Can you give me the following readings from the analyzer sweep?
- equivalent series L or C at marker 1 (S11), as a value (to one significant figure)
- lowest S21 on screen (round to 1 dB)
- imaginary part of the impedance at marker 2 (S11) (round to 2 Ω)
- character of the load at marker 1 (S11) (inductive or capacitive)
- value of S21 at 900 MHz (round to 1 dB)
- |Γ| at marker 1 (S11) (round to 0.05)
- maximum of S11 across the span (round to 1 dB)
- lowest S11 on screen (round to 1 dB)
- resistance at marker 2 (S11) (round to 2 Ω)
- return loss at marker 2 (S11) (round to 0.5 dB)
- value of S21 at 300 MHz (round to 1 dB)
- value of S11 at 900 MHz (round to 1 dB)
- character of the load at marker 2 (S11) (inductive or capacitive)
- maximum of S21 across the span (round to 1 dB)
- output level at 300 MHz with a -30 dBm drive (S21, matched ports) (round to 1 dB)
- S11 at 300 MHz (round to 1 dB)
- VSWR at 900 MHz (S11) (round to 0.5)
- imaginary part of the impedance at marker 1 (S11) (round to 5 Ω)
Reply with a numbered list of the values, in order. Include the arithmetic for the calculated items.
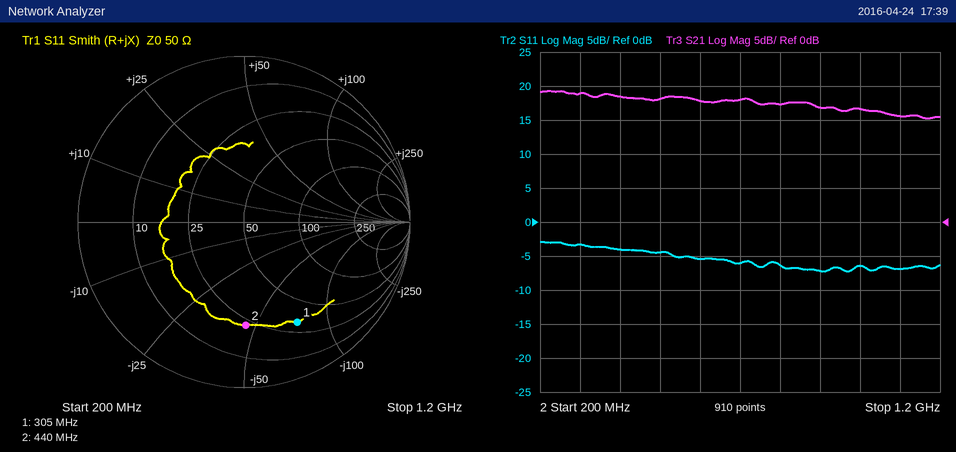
1. C = 1/(2π × 305 MHz × 75 Ω) ≈ 7 pF
2. 15 dB
3. -46 Ω
4. capacitive
5. 17 dB
6. 0.70
7. -3 dB
8. -7 dB
9. 22 Ω
10. 4.0 dB
11. 19 dB
12. -7 dB
13. capacitive
14. 19 dB
15. -30 dBm + (19 dB) = -11 dBm
16. -3 dB
17. |Γ| = 10^(-7/20) = 0.4467; VSWR = (1 + 0.4467)/(1 − 0.4467) ≈ 2.61, so 2.5 to the nearest 0.5
18. -75 Ω
